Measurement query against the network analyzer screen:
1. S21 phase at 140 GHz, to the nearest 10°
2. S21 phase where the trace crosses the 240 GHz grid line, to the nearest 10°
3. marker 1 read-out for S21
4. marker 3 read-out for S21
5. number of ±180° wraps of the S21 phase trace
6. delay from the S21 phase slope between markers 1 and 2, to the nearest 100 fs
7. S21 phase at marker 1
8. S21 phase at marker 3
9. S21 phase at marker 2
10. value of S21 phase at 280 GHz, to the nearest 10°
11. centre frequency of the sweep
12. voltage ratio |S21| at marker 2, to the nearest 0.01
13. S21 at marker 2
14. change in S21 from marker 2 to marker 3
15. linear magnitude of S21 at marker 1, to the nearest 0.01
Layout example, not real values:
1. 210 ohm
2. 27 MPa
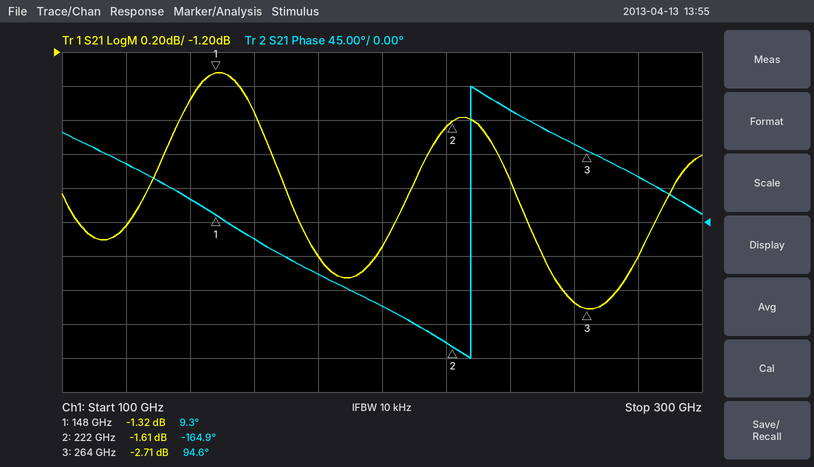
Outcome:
1. 30°
2. 150°
3. -1.32 dB
4. -2.71 dB
5. 1
6. 6.5 ps
7. 9.3°
8. 94.6°
9. -164.9°
10. 60°
11. 200 GHz
12. 0.83
13. -1.61 dB
14. -1.10 dB
15. 0.86
